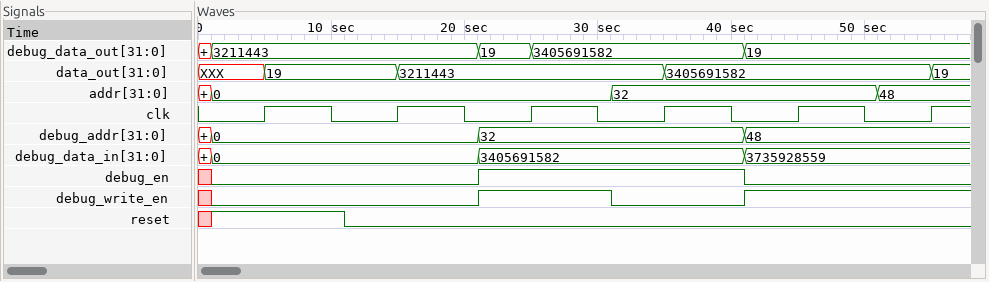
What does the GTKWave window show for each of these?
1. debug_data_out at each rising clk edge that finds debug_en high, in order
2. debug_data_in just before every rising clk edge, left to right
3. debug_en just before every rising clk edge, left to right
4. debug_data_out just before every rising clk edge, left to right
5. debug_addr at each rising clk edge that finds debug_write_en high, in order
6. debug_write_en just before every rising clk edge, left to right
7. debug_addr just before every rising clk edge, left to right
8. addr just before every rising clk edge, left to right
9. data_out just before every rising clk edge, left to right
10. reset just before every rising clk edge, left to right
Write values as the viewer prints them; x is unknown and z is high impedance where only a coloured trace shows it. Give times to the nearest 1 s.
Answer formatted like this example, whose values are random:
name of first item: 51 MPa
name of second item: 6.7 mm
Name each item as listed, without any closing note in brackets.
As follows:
debug_data_out at each rising clk edge that finds debug_en high, in order: 19, 3405691582
debug_data_in just before every rising clk edge, left to right: 0, 0, 3405691582, 3405691582, 3735928559, 3735928559
debug_en just before every rising clk edge, left to right: 0 0 1 1 0 0
debug_data_out just before every rising clk edge, left to right: 3211443, 3211443, 19, 3405691582, 19, 19
debug_addr at each rising clk edge that finds debug_write_en high, in order: 32, 48, 48
debug_write_en just before every rising clk edge, left to right: 0 0 1 0 1 1
debug_addr just before every rising clk edge, left to right: 0, 0, 32, 32, 48, 48
addr just before every rising clk edge, left to right: 0, 0, 0, 32, 32, 48
data_out just before every rising clk edge, left to right: XXX, 19, 3211443, 3211443, 3405691582, 3405691582
reset just before every rising clk edge, left to right: 1 0 0 0 0 0
